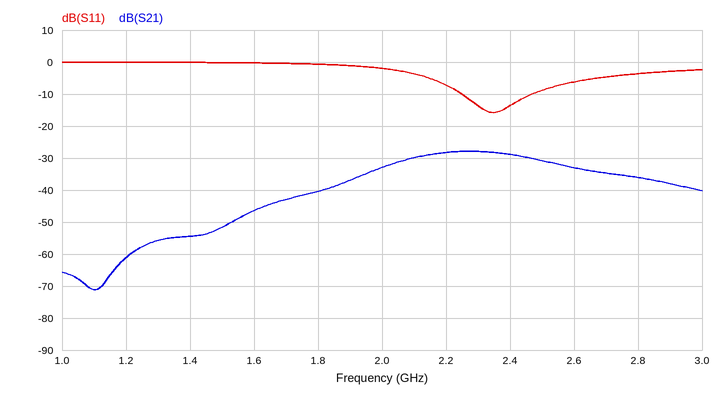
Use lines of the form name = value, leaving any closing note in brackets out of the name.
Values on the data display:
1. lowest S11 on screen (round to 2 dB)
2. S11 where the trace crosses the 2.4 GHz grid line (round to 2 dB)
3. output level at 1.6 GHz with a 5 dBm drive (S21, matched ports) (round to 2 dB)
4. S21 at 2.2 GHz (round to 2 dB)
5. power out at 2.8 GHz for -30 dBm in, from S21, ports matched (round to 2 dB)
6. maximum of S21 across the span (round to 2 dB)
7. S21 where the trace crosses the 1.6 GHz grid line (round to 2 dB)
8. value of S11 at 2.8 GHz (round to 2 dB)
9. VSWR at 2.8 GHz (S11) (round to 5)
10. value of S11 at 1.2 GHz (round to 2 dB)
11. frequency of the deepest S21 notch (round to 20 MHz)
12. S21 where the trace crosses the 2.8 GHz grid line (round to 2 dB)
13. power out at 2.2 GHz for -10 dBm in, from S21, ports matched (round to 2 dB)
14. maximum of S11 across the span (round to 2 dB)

lowest S11 on screen = -16 dB
S11 where the trace crosses the 2.4 GHz grid line = -14 dB
output level at 1.6 GHz with a 5 dBm drive (S21, matched ports) = -42 dBm
S21 at 2.2 GHz = -28 dB
power out at 2.8 GHz for -30 dBm in, from S21, ports matched = -66 dBm
maximum of S21 across the span = -28 dB
S21 where the trace crosses the 1.6 GHz grid line = -46 dB
value of S11 at 2.8 GHz = -4 dB
VSWR at 2.8 GHz (S11) = 5
value of S11 at 1.2 GHz = 0 dB
frequency of the deepest S21 notch = 1.10 GHz
S21 where the trace crosses the 2.8 GHz grid line = -36 dB
power out at 2.2 GHz for -10 dBm in, from S21, ports matched = -38 dBm
maximum of S11 across the span = 0 dB
